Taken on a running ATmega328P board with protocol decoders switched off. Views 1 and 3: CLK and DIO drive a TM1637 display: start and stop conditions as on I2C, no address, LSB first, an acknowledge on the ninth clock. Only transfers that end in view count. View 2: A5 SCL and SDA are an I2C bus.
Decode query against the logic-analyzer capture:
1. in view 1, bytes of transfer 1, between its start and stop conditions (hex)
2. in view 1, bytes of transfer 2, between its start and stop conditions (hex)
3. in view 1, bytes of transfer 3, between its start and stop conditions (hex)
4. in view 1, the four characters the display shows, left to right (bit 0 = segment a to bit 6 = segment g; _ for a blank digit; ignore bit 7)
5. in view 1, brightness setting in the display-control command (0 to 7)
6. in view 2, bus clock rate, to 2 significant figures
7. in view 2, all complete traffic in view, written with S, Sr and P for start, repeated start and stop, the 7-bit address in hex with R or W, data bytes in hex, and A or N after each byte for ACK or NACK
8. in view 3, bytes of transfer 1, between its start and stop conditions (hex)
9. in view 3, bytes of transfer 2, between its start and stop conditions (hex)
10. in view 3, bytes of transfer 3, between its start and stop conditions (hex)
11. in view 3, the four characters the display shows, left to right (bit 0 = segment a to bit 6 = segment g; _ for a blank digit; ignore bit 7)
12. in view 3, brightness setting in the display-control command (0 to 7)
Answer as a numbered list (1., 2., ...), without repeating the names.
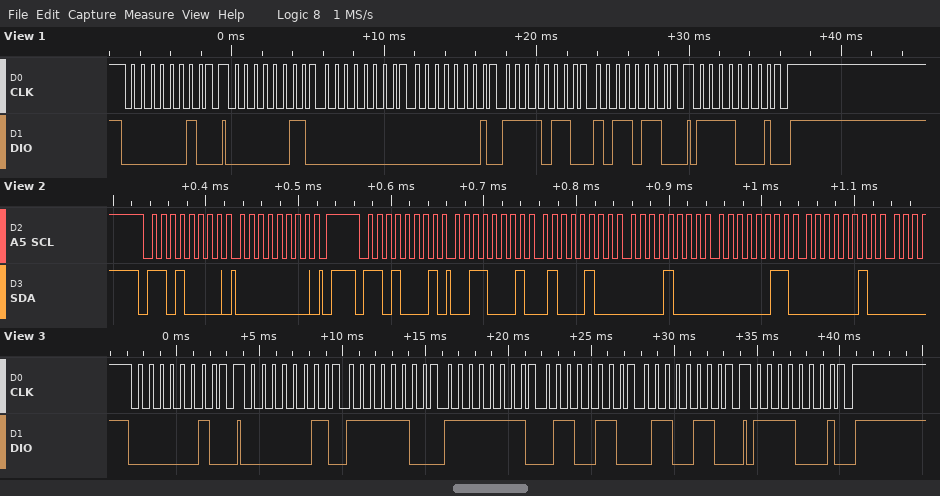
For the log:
1. 40
2. C0 00 80 6F 6D
3. 8F
4. __95
5. 7
6. 100 kHz
7. S 68W A 00 A P S 68R A 31 A 44 A 08 A 03 A 02 A
8. 40
9. C0 3F FF 66 66
10. 8F
11. 0844
12. 7
